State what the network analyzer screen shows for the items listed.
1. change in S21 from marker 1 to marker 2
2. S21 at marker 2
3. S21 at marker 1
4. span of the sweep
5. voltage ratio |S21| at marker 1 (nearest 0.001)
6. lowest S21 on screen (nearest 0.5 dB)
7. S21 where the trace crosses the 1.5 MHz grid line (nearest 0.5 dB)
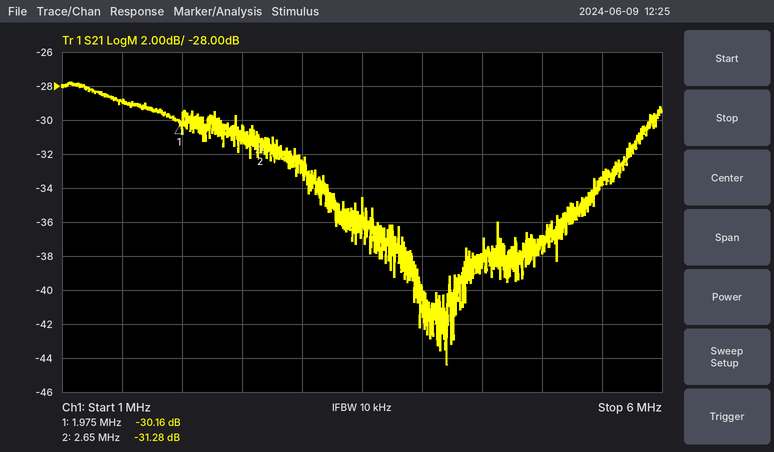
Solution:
-1.12 dB
-31.28 dB
-30.16 dB
5 MHz
0.031
-44.5 dB
-29.0 dB
